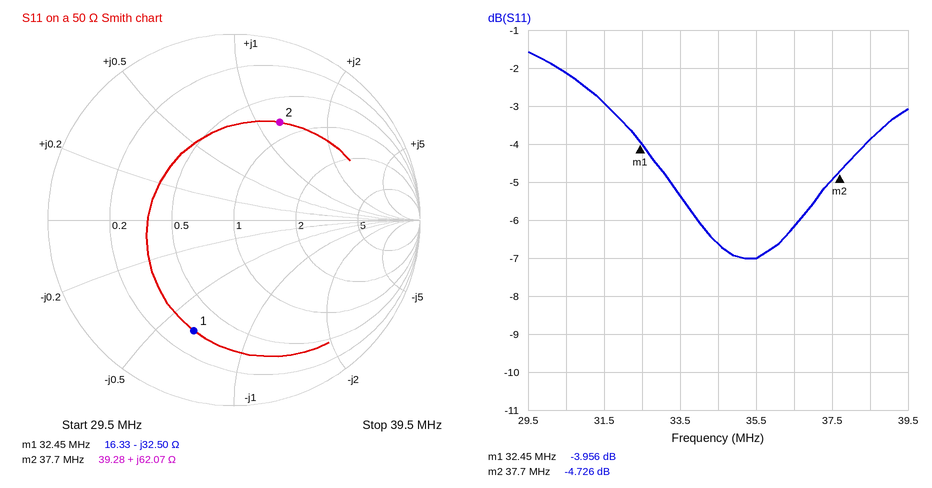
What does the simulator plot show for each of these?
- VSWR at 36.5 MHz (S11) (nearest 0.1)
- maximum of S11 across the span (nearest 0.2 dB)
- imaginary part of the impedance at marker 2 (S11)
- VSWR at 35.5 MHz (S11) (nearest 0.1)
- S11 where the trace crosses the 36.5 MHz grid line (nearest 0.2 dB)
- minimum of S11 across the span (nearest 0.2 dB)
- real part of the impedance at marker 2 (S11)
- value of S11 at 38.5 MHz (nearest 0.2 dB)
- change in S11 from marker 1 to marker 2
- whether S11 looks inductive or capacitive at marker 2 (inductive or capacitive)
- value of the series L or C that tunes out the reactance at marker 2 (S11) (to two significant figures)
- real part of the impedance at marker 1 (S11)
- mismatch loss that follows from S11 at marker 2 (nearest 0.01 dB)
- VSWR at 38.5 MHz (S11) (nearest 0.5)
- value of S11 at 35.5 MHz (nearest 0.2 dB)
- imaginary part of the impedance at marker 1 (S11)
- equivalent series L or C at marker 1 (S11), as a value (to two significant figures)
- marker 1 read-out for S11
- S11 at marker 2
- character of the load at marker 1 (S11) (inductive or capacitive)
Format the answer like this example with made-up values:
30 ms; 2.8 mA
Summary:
2.9; -1.6 dB; +62.07 Ω; 2.6; -6.2 dB; -7.0 dB; 39.28 Ω; -3.8 dB; -0.770 dB; inductive; 68 pF; 16.33 Ω; 1.78 dB; 4.5; -7.0 dB; -32.50 Ω; 150 pF; -3.956 dB; -4.726 dB; capacitive
